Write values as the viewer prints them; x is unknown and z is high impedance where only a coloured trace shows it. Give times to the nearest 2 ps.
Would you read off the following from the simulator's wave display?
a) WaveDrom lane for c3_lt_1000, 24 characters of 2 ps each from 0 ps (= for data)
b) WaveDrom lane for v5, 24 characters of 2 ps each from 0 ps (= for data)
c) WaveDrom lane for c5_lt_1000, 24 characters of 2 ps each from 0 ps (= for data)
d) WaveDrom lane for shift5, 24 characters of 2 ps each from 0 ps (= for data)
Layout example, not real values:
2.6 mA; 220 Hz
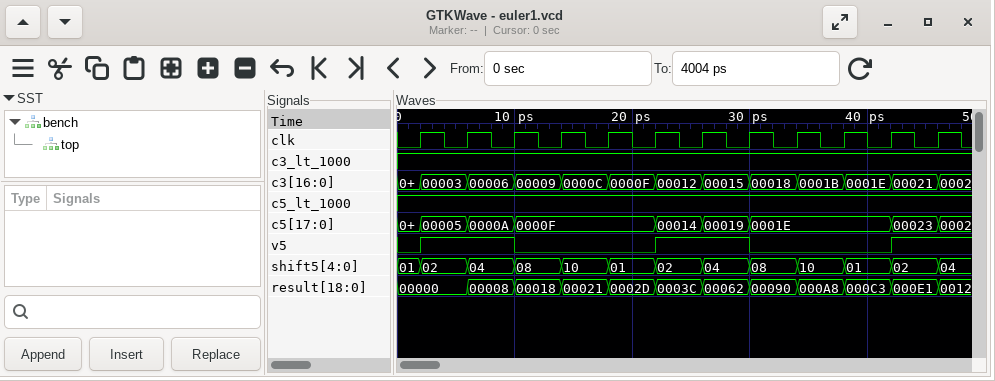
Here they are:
{name: 'c3_lt_1000', wave: '1.......................'}; {name: 'v5', wave: '01...0.....1...0.....1..'}; {name: 'c5_lt_1000', wave: '1.......................'}; {name: 'shift5', wave: '==.=.=.=.=.=.=.=.=.=.=.=', data: '01 02 04 08 10 01 02 04 08 10 01 02 04'}
